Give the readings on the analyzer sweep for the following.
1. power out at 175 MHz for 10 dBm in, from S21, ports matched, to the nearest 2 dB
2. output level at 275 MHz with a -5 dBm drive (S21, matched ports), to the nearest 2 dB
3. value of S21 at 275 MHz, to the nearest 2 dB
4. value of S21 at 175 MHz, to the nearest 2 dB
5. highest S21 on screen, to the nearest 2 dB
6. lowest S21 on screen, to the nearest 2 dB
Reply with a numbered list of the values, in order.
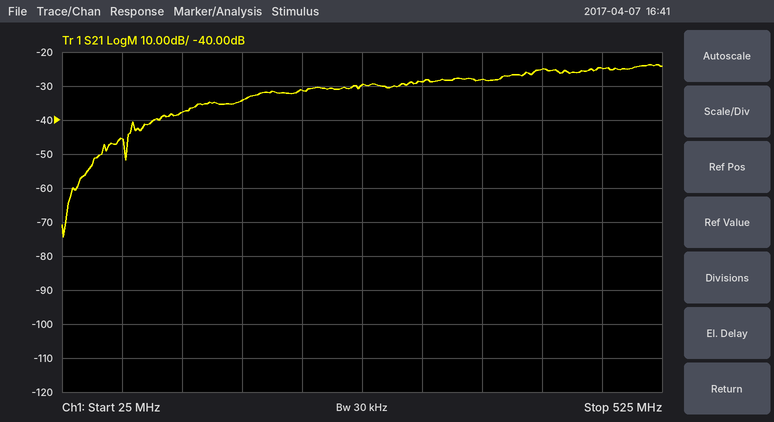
1. -24 dBm
2. -34 dBm
3. -30 dB
4. -34 dB
5. -24 dB
6. -74 dB
